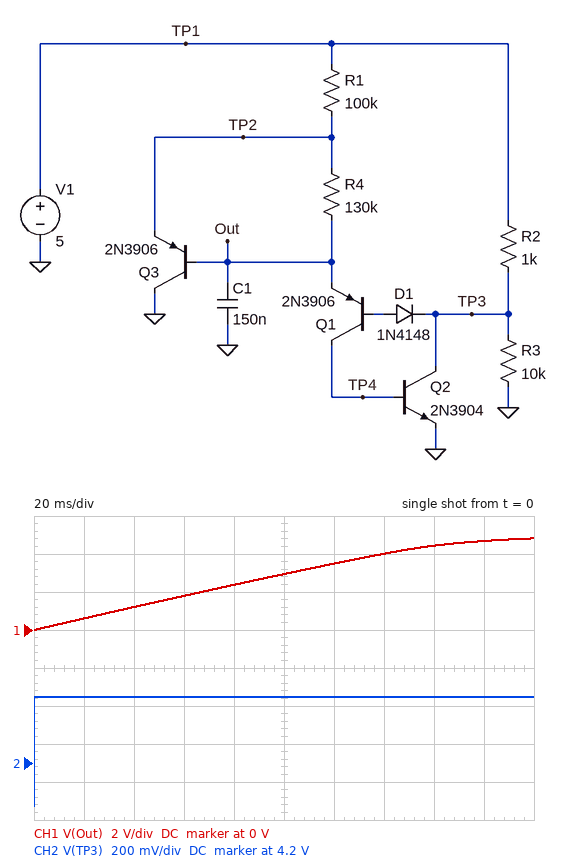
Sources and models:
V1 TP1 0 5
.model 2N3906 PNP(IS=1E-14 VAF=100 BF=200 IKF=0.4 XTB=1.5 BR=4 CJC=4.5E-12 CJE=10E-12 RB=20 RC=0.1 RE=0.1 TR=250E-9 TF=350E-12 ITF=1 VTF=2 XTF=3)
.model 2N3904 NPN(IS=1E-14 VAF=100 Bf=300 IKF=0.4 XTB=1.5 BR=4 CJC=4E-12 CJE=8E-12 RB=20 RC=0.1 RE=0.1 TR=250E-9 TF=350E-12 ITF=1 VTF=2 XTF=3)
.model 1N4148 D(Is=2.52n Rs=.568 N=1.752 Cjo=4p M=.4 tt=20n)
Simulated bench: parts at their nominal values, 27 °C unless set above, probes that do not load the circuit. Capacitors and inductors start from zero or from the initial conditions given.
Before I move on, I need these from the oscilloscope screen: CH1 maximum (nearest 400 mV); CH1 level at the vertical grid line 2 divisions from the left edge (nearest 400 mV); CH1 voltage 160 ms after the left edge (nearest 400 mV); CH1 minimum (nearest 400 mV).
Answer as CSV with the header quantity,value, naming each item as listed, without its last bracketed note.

quantity,value
CH1 maximum,4.8 V
CH1 level at the vertical grid line 2 divisions from the left edge,1.2 V
CH1 voltage 160 ms after the left edge,4.4 V
CH1 minimum,0 V
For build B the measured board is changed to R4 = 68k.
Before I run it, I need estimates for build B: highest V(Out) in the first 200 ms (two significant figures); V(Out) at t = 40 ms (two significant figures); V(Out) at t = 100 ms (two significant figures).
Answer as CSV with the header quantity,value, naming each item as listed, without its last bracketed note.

quantity,value
highest V(Out) in the first 200 ms,4.9 V
V(Out) at t = 40 ms,2.2 V
V(Out) at t = 100 ms,4.6 V
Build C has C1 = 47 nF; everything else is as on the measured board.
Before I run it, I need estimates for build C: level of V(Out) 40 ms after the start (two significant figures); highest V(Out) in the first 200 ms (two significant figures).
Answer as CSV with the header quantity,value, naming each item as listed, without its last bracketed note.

quantity,value
level of V(Out) 40 ms after the start,3.7 V
highest V(Out) in the first 200 ms,4.9 V
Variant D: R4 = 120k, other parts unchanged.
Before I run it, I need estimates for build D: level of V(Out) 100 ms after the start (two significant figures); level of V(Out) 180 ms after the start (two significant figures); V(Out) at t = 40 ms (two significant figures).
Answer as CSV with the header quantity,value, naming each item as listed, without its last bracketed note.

quantity,value
level of V(Out) 100 ms after the start,3.2 V
level of V(Out) 180 ms after the start,4.8 V
V(Out) at t = 40 ms,1.3 V
